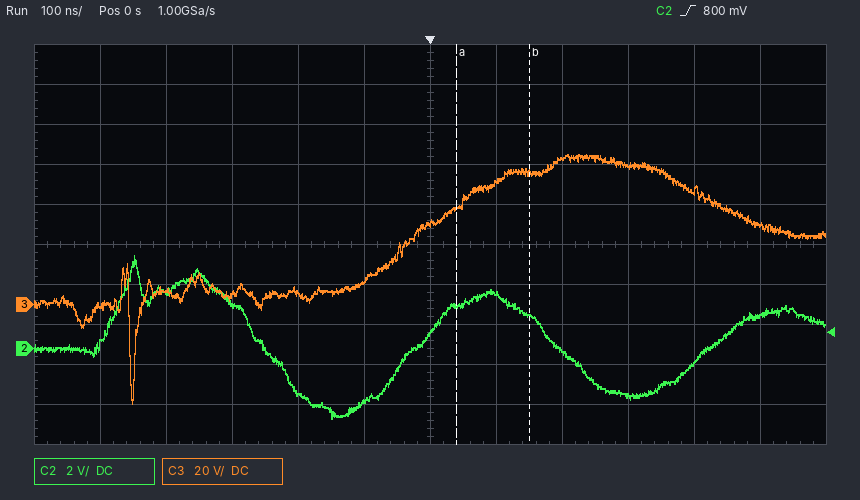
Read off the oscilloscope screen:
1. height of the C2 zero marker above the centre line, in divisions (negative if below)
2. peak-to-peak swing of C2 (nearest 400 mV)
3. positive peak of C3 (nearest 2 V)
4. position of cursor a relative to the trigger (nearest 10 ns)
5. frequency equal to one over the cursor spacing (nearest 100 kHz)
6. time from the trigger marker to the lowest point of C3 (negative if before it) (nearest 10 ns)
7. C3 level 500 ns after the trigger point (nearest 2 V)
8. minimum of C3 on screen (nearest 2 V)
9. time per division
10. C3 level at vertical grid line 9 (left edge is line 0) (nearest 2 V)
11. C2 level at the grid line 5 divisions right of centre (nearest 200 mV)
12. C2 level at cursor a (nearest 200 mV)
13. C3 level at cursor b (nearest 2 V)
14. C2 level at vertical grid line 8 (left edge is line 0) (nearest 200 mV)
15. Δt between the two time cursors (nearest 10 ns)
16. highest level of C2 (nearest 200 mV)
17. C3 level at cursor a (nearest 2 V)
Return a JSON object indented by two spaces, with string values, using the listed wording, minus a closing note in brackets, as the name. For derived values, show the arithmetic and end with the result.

{
  "height of the C2 zero marker above the centre line, in divisions": "-2.6 div",
  "peak-to-peak swing of C2": "8.0 V",
  "positive peak of C3": "76 V",
  "position of cursor a relative to the trigger": "+40 ns",
  "frequency equal to one over the cursor spacing": "1 / 110 ns ≈ 9.1 MHz",
  "time from the trigger marker to the lowest point of C3 (negative if before it)": "-450 ns",
  "C3 level 500 ns after the trigger point": "40 V",
  "minimum of C3 on screen": "-50 V",
  "time per division": "100 ns",
  "C3 level at vertical grid line 9 (left edge is line 0)": "70 V",
  "C2 level at the grid line 5 divisions right of centre": "1.6 V",
  "C2 level at cursor a": "2.2 V",
  "C3 level at cursor b": "66 V",
  "C2 level at vertical grid line 8 (left edge is line 0)": "-200 mV",
  "Δt between the two time cursors": "110 ns",
  "highest level of C2": "4.6 V",
  "C3 level at cursor a": "48 V"
}
